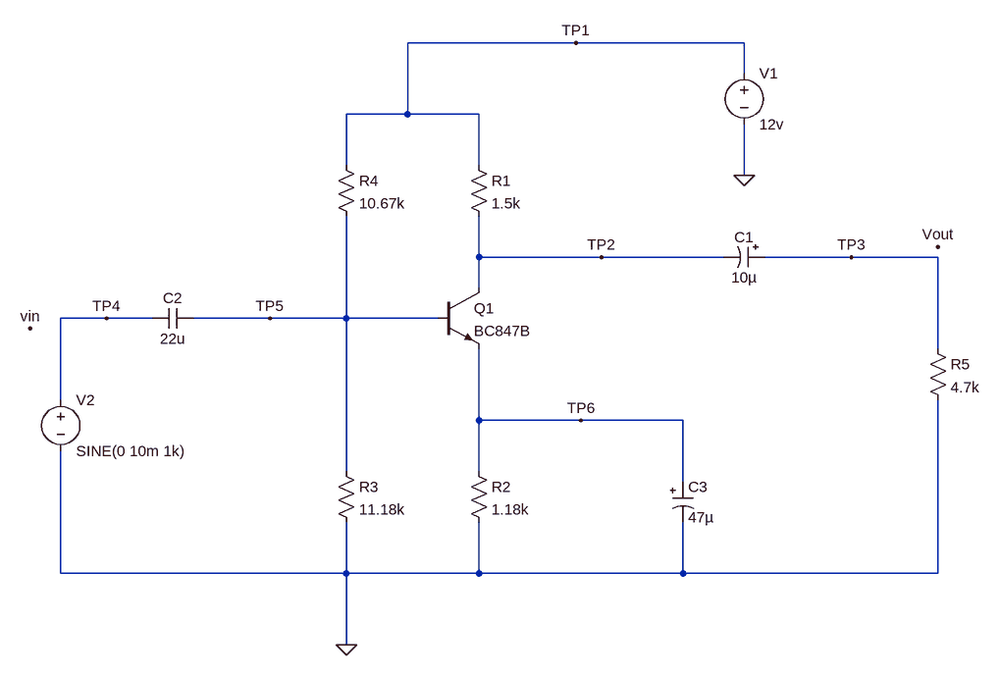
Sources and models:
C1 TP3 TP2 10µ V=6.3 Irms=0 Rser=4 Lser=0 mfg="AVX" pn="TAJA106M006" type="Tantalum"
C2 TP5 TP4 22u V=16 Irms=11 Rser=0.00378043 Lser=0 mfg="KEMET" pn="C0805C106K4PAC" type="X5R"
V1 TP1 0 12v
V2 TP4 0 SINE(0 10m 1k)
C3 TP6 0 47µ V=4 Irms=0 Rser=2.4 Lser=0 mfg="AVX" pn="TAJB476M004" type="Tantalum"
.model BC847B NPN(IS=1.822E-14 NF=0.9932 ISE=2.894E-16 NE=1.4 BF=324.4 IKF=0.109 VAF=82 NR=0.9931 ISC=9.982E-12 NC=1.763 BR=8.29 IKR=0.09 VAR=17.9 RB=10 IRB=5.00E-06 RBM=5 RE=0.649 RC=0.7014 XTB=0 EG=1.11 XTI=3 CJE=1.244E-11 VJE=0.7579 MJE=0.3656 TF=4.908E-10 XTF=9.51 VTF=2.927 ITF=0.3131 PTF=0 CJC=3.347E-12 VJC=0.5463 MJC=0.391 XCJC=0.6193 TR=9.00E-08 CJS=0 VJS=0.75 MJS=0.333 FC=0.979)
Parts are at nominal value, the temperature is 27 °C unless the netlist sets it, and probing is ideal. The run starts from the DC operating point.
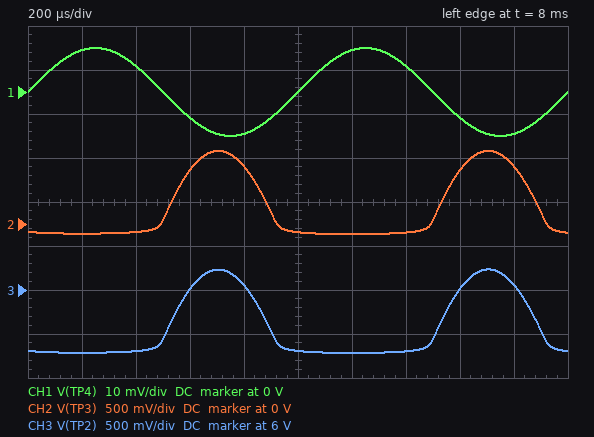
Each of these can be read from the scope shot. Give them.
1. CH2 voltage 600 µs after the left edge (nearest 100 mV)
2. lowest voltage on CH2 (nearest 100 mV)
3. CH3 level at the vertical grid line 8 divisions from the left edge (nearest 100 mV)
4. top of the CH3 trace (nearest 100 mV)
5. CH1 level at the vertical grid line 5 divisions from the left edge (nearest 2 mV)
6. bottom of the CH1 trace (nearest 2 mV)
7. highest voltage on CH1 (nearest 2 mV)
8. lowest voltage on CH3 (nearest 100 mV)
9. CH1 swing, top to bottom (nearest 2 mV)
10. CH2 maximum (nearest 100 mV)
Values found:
600 mV
-100 mV
6.0 V
6.2 V
0 V
-10 mV
10 mV
5.3 V
20 mV
800 mV
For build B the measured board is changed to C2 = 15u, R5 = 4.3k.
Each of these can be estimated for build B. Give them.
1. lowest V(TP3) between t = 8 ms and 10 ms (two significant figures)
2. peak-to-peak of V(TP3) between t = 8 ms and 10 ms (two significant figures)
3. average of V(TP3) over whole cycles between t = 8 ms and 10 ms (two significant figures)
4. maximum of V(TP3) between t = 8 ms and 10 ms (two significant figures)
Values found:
-130 mV
980 mV
190 mV
860 mV
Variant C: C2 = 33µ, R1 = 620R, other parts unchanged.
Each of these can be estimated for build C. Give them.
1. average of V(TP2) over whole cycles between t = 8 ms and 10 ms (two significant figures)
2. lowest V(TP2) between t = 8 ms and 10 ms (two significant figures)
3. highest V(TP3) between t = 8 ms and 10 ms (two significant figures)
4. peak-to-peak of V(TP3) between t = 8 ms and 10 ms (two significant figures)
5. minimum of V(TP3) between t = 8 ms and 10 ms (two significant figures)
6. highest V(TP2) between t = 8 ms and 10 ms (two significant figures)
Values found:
9.2 V
8.6 V
540 mV
1.1 V
-580 mV
9.7 V
